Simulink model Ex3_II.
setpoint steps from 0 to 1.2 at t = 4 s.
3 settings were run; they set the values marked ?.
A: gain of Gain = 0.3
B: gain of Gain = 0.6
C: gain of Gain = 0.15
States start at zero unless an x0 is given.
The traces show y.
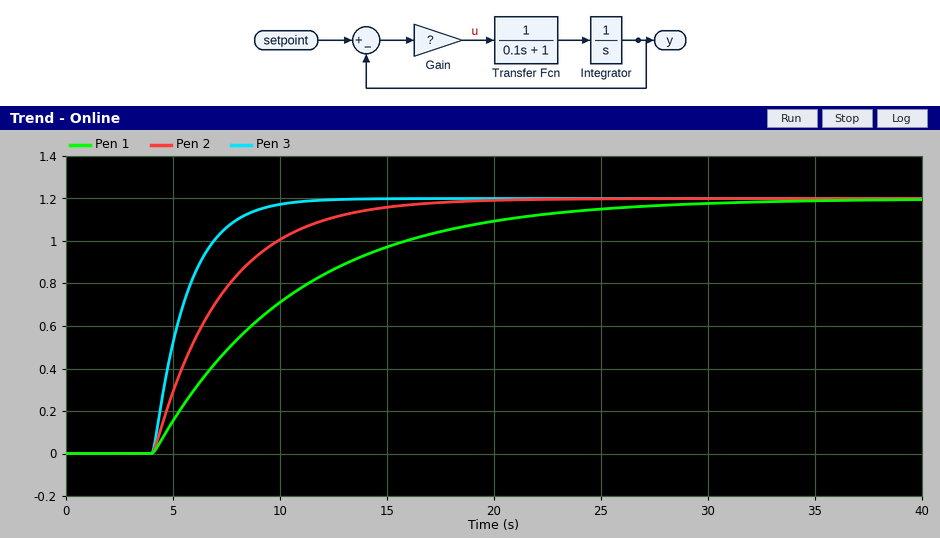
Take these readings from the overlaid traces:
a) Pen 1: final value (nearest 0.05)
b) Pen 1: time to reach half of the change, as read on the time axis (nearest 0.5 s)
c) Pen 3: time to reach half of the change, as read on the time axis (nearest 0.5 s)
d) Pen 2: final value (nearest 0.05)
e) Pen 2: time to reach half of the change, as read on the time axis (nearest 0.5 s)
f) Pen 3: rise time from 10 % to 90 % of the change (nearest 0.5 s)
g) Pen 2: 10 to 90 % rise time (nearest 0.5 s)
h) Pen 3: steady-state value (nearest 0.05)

1.20
8.5 s
5.0 s
1.20
6.5 s
3.5 s
7.0 s
1.20
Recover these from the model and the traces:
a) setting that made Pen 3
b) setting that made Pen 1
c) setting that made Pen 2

B
C
A
